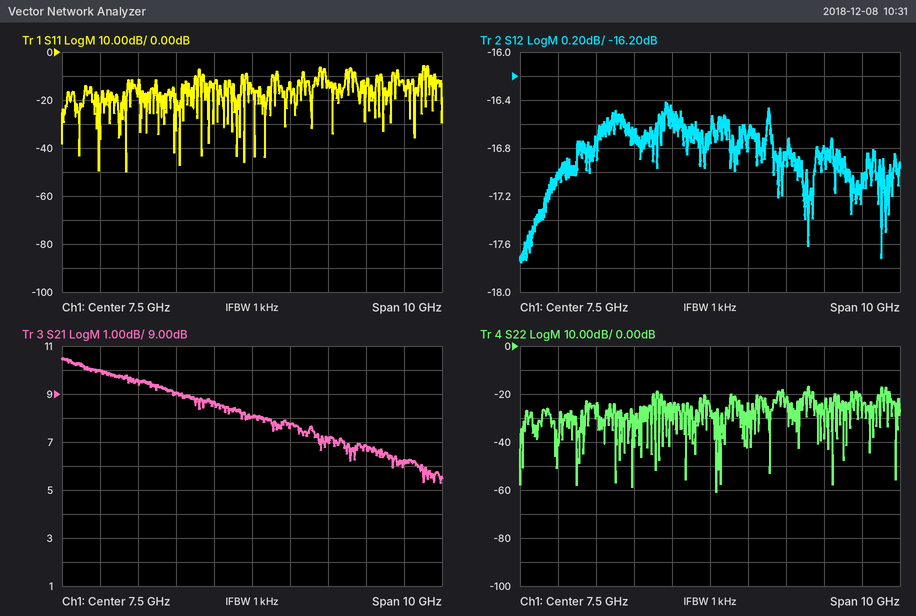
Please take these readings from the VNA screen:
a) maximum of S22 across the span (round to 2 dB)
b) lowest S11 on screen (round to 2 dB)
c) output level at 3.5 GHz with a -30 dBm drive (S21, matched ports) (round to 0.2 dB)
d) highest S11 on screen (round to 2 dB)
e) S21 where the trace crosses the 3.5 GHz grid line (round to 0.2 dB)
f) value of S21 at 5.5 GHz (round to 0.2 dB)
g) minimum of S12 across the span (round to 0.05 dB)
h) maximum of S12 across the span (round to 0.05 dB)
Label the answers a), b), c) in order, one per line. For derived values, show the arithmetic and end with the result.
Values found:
a) -16 dB
b) -50 dB
c) -30 dBm + (10.0 dB) = -20.0 dBm
d) -6 dB
e) 10.0 dB
f) 9.0 dB
g) -17.75 dB
h) -16.40 dB
